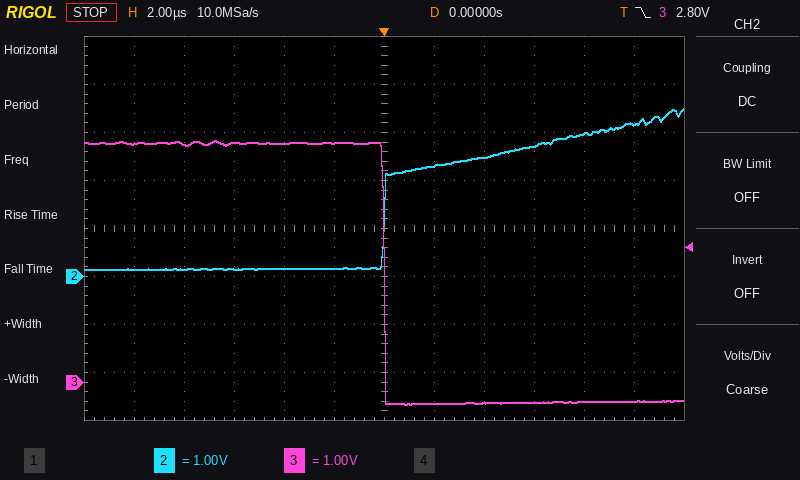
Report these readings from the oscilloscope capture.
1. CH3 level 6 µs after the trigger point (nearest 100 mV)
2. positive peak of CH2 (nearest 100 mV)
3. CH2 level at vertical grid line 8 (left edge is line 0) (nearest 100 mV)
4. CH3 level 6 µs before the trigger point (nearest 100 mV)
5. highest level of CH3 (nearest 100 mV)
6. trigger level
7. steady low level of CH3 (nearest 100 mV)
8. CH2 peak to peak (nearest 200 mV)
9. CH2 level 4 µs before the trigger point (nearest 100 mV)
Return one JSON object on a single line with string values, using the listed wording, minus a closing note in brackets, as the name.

{"CH3 level 6 µs after the trigger point": "-400 mV", "positive peak of CH2": "3.5 V", "CH2 level at vertical grid line 8 (left edge is line 0)": "2.5 V", "CH3 level 6 µs before the trigger point": "5.0 V", "highest level of CH3": "5.0 V", "trigger level": "2.80 V", "steady low level of CH3": "-400 mV", "CH2 peak to peak": "3.4 V", "CH2 level 4 µs before the trigger point": "200 mV"}
